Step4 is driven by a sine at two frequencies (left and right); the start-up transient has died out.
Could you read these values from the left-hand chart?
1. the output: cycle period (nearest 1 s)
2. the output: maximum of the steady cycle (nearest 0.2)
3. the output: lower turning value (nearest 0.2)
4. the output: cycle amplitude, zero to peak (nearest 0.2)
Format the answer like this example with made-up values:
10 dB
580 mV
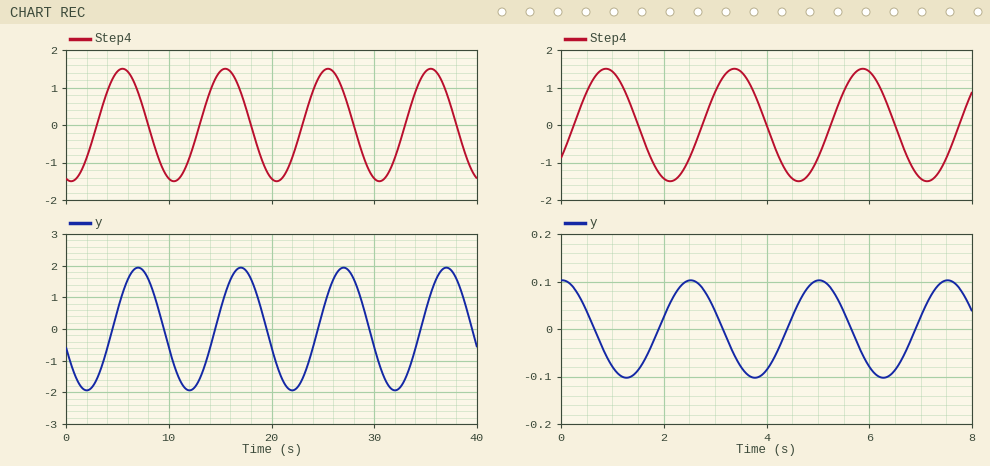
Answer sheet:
10 s
2.0
-2.0
2.0
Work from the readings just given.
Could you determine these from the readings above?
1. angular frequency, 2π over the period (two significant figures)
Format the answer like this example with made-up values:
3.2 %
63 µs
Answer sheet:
0.63 rad/s
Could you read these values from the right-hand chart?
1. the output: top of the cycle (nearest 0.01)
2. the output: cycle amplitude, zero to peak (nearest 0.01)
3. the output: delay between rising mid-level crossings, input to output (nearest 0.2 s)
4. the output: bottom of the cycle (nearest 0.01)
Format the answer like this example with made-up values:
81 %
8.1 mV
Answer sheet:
0.10
0.10
1.6 s
-0.10
